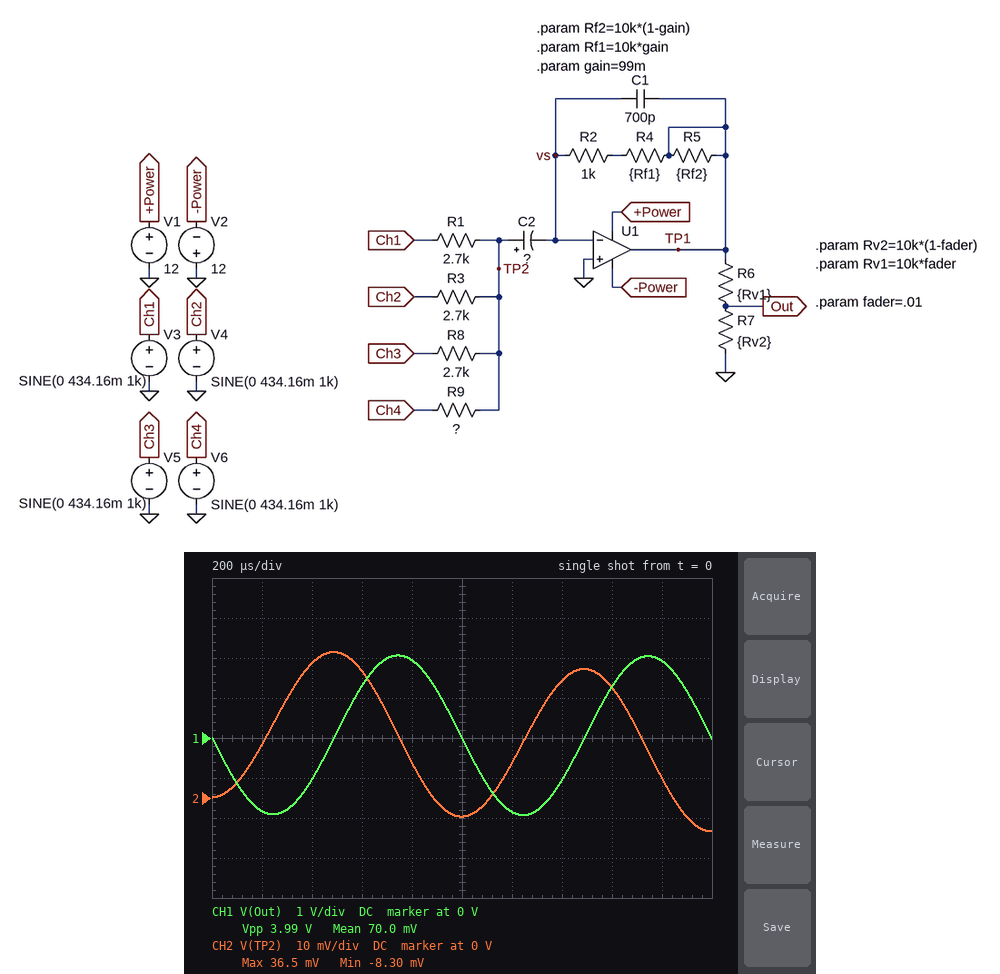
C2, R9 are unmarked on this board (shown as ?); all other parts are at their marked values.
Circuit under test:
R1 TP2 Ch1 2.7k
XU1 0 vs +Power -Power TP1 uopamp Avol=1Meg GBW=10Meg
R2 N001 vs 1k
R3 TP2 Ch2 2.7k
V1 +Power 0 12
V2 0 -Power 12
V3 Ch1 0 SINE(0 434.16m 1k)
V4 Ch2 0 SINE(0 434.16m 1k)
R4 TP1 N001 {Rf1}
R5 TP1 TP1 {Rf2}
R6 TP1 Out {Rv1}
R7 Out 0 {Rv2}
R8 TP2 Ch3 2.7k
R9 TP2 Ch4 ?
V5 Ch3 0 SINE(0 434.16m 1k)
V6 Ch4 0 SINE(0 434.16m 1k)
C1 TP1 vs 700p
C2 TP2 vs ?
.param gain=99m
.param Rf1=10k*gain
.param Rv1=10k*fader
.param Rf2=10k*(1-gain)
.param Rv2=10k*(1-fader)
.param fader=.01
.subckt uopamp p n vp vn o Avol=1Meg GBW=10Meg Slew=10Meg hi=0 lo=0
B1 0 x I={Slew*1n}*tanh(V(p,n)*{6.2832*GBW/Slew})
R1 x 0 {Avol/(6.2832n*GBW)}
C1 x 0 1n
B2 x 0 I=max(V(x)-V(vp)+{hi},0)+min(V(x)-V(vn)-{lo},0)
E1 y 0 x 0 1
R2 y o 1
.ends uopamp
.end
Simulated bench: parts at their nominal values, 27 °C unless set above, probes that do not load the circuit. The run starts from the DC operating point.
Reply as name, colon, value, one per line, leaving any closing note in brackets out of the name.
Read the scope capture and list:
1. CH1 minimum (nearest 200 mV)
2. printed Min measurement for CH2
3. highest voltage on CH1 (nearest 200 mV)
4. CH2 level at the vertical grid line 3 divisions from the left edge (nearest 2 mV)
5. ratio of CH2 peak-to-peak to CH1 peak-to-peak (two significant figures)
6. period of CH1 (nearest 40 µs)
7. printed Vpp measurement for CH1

CH1 minimum: -2.0 V
printed Min measurement for CH2: -8.30 mV
highest voltage on CH1: 2.0 V
CH2 level at the vertical grid line 3 divisions from the left edge: 32 mV
ratio of CH2 peak-to-peak to CH1 peak-to-peak: 0.011
period of CH1: 1.00 ms
printed Vpp measurement for CH1: 3.99 V
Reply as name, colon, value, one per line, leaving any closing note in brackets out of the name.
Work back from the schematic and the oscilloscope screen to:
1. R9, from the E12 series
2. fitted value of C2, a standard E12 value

R9, from the E12 series: 820 Ω
fitted value of C2, a standard E12 value: 8.2 µF
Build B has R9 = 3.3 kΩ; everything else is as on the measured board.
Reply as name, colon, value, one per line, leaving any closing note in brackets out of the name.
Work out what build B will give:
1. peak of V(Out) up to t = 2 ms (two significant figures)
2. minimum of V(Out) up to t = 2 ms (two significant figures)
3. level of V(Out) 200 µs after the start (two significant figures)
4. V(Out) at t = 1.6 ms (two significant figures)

peak of V(Out) up to t = 2 ms: 1.2 V
minimum of V(Out) up to t = 2 ms: -1.2 V
level of V(Out) 200 µs after the start: -1.1 V
V(Out) at t = 1.6 ms: 750 mV
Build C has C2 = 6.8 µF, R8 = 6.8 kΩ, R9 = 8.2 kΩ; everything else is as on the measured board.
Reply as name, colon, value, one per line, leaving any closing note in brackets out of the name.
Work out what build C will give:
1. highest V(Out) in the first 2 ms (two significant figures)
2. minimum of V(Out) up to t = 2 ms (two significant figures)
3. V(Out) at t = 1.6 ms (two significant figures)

highest V(Out) in the first 2 ms: 880 mV
minimum of V(Out) up to t = 2 ms: -850 mV
V(Out) at t = 1.6 ms: 530 mV
